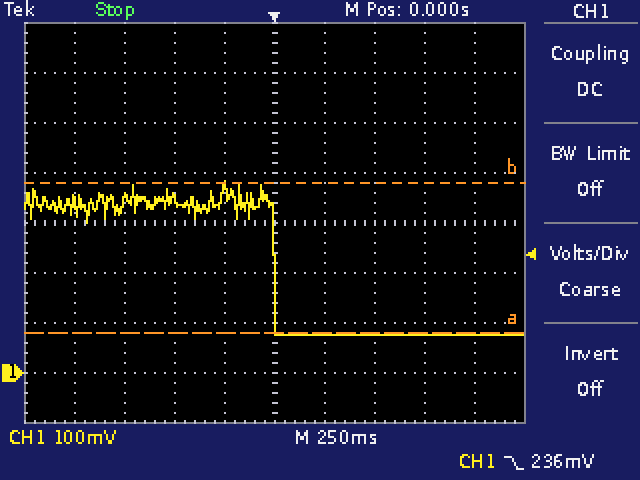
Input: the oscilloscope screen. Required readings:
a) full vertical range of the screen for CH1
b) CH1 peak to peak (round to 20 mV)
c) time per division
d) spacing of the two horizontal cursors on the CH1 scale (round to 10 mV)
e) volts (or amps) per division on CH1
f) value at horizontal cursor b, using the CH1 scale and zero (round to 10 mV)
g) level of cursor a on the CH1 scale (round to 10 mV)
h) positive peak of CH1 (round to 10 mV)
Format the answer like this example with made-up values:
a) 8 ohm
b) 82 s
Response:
a) 800 mV
b) 300 mV
c) 250 ms
d) 300 mV
e) 100 mV
f) 380 mV
g) 80 mV
h) 380 mV
